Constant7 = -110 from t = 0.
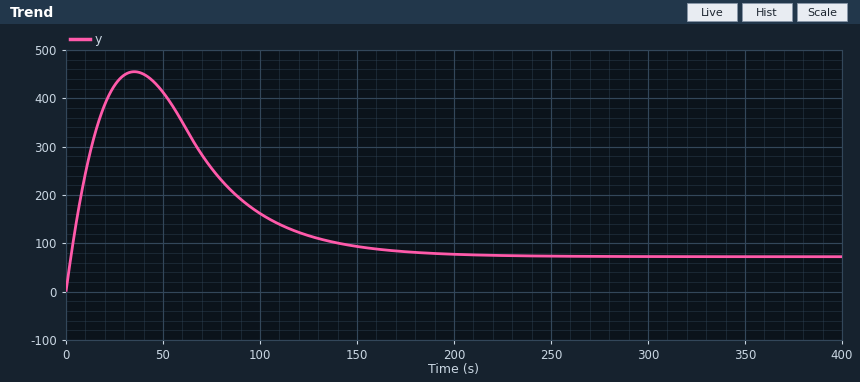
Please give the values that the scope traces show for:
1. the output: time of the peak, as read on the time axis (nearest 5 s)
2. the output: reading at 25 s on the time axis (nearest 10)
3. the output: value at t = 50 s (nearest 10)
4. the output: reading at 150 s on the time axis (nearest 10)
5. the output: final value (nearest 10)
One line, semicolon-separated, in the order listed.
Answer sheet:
35 s; 430; 410; 90; 70
